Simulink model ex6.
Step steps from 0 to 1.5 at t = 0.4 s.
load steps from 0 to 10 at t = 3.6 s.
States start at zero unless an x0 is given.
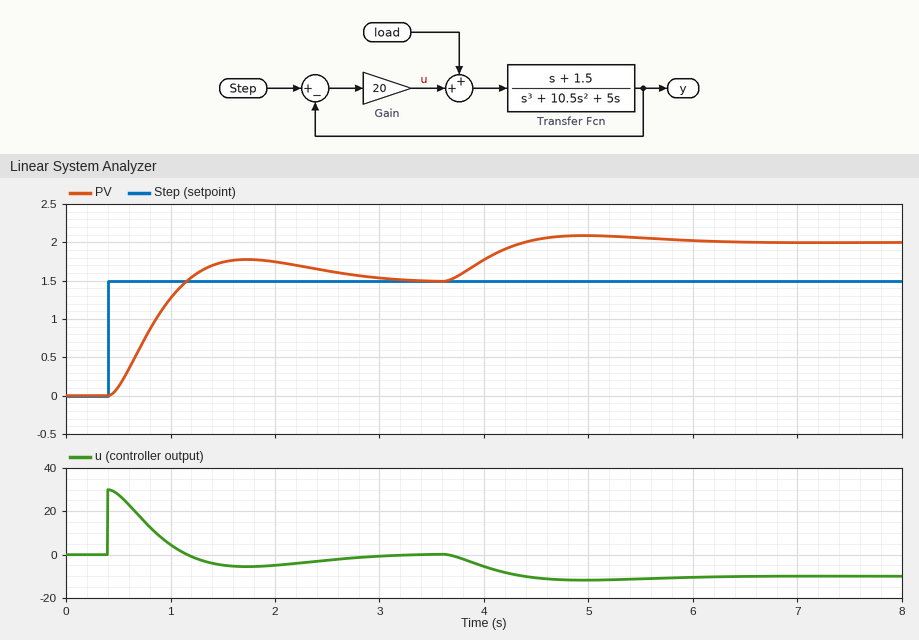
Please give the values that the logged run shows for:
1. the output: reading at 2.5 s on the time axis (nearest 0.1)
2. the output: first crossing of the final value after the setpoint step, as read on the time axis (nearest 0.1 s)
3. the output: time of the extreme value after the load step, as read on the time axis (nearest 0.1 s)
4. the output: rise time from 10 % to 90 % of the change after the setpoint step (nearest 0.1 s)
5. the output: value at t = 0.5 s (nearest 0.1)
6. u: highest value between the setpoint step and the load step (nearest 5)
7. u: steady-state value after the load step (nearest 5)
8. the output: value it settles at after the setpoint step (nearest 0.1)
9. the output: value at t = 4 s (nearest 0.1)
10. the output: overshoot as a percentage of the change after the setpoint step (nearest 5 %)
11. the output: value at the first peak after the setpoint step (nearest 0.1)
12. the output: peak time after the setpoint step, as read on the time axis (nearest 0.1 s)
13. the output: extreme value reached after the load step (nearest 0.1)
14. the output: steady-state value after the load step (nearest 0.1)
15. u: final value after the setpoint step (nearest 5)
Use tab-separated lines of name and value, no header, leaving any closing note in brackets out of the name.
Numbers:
the output: reading at 2.5 s on the time axis	1.6
the output: first crossing of the final value after the setpoint step, as read on the time axis	1.2 s
the output: time of the extreme value after the load step, as read on the time axis	5.0 s
the output: rise time from 10 % to 90 % of the change after the setpoint step	0.5 s
the output: value at t = 0.5 s	0.1
u: highest value between the setpoint step and the load step	30
u: steady-state value after the load step	-10
the output: value it settles at after the setpoint step	1.5
the output: value at t = 4 s	1.8
the output: overshoot as a percentage of the change after the setpoint step	20 %
the output: value at the first peak after the setpoint step	1.8
the output: peak time after the setpoint step, as read on the time axis	1.7 s
the output: extreme value reached after the load step	2.1
the output: steady-state value after the load step	2.0
u: final value after the setpoint step	0
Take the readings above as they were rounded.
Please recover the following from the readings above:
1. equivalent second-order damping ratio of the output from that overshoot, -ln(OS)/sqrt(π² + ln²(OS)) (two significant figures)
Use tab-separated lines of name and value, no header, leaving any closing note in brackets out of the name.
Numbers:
equivalent second-order damping ratio of the output from that overshoot, -ln(OS)/sqrt(π² + ln²(OS))	0.46
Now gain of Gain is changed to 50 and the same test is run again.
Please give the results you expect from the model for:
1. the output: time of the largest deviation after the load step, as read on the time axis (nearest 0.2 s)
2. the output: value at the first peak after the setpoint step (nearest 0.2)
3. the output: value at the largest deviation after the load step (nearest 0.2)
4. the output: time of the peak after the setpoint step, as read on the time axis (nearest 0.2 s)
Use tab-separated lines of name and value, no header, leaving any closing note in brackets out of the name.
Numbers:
the output: time of the largest deviation after the load step, as read on the time axis	4.2 s
the output: value at the first peak after the setpoint step	1.8
the output: value at the largest deviation after the load step	1.8
the output: time of the peak after the setpoint step, as read on the time axis	1.0 s
